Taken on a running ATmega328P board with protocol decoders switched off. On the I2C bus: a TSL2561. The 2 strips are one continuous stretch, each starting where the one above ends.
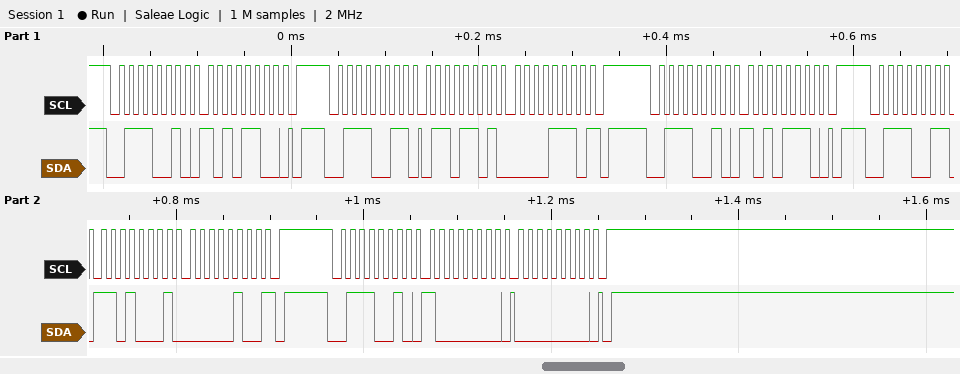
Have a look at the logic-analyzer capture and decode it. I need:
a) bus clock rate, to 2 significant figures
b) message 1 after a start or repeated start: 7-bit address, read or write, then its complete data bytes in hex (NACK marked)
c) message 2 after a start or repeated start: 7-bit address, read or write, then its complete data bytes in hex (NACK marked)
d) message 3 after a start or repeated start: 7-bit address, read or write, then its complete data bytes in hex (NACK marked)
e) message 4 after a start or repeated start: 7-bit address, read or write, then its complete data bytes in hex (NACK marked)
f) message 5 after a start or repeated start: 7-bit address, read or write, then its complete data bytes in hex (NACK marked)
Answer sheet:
100 kHz
0x39 write: AC
0x39 read: 6D 0E NACK
0x39 write: AE
0x39 read: D1 04 NACK
0x39 write: 80 00
